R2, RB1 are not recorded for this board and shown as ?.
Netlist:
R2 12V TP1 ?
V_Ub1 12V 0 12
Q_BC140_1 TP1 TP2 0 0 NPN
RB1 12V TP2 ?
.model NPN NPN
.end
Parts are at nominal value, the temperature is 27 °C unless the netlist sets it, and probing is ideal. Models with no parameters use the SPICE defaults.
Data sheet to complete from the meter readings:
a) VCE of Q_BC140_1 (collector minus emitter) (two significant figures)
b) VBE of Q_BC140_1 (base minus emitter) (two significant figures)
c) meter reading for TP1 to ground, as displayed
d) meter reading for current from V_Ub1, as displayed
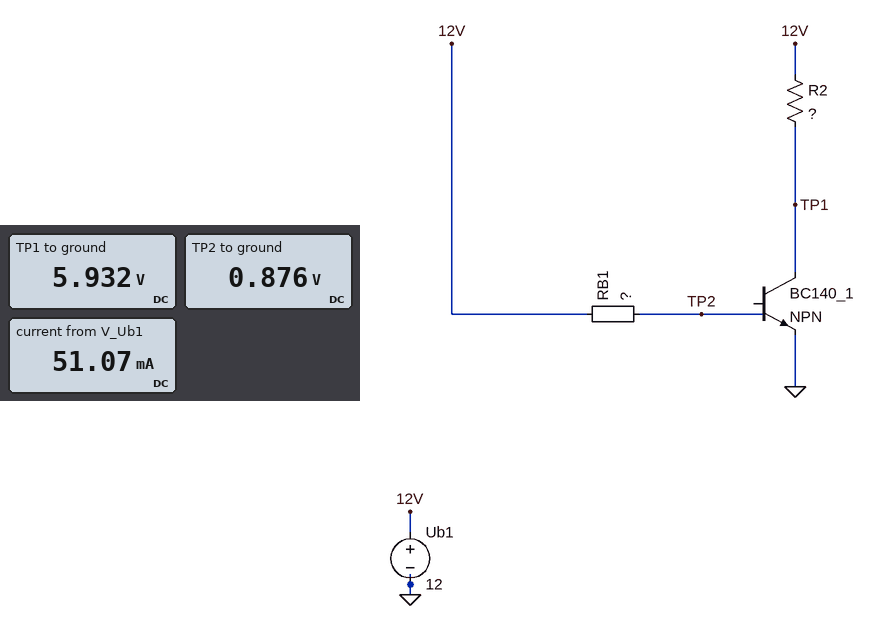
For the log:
5.9 V
880 mV
5.932 V
51.07 mA
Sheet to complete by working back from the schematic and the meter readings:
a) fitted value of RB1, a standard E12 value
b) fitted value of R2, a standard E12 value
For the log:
22 kΩ
120 Ω
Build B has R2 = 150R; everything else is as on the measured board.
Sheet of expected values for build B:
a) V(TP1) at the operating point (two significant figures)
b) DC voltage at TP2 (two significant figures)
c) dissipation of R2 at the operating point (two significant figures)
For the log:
4.4 V
880 mV
380 mW
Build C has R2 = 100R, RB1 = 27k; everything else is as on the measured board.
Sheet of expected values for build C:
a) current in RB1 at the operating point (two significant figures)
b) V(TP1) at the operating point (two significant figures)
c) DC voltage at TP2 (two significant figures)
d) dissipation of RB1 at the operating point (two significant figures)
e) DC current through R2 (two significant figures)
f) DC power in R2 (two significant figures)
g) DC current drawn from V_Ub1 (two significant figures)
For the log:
410 µA
7.9 V
870 mV
4.6 mW
41 mA
170 mW
42 mA
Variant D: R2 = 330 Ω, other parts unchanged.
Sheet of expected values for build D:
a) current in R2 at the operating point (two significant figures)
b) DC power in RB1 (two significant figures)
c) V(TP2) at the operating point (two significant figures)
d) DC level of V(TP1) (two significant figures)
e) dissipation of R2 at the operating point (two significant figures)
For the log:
36 mA
5.6 mW
870 mV
140 mV
430 mW
